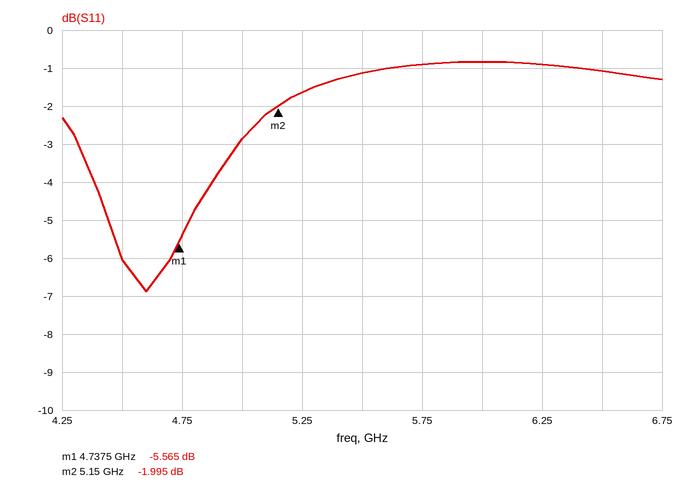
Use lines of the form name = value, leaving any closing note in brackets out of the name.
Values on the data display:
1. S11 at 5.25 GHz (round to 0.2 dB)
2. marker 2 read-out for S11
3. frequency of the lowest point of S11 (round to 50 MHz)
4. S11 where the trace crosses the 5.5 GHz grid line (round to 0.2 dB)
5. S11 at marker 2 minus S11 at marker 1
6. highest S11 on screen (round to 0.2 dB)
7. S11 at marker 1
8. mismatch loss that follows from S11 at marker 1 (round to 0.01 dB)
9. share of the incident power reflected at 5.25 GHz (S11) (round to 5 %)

S11 at 5.25 GHz = -1.6 dB
marker 2 read-out for S11 = -1.995 dB
frequency of the lowest point of S11 = 4.60 GHz
S11 where the trace crosses the 5.5 GHz grid line = -1.2 dB
S11 at marker 2 minus S11 at marker 1 = 3.570 dB
highest S11 on screen = -0.8 dB
S11 at marker 1 = -5.565 dB
mismatch loss that follows from S11 at marker 1 = 1.41 dB
share of the incident power reflected at 5.25 GHz (S11) = 70 %
